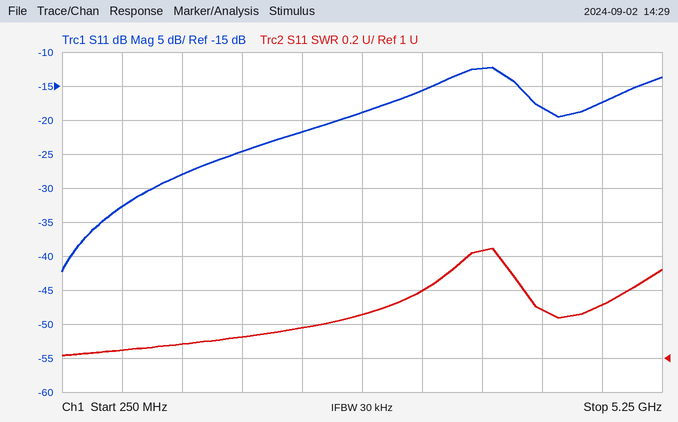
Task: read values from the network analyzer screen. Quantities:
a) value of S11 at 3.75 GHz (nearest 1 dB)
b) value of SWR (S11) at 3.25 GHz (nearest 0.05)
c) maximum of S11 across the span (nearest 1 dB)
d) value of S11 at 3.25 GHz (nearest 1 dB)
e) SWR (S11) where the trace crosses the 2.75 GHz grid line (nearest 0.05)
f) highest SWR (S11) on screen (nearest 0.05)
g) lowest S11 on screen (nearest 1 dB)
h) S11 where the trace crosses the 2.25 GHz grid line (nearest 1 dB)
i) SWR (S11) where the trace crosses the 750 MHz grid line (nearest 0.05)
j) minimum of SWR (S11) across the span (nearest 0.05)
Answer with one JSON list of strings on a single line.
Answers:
["-12 dB", "1.40", "-12 dB", "-16 dB", "1.25", "1.65", "-42 dB", "-22 dB", "1.05", "1.00"]
